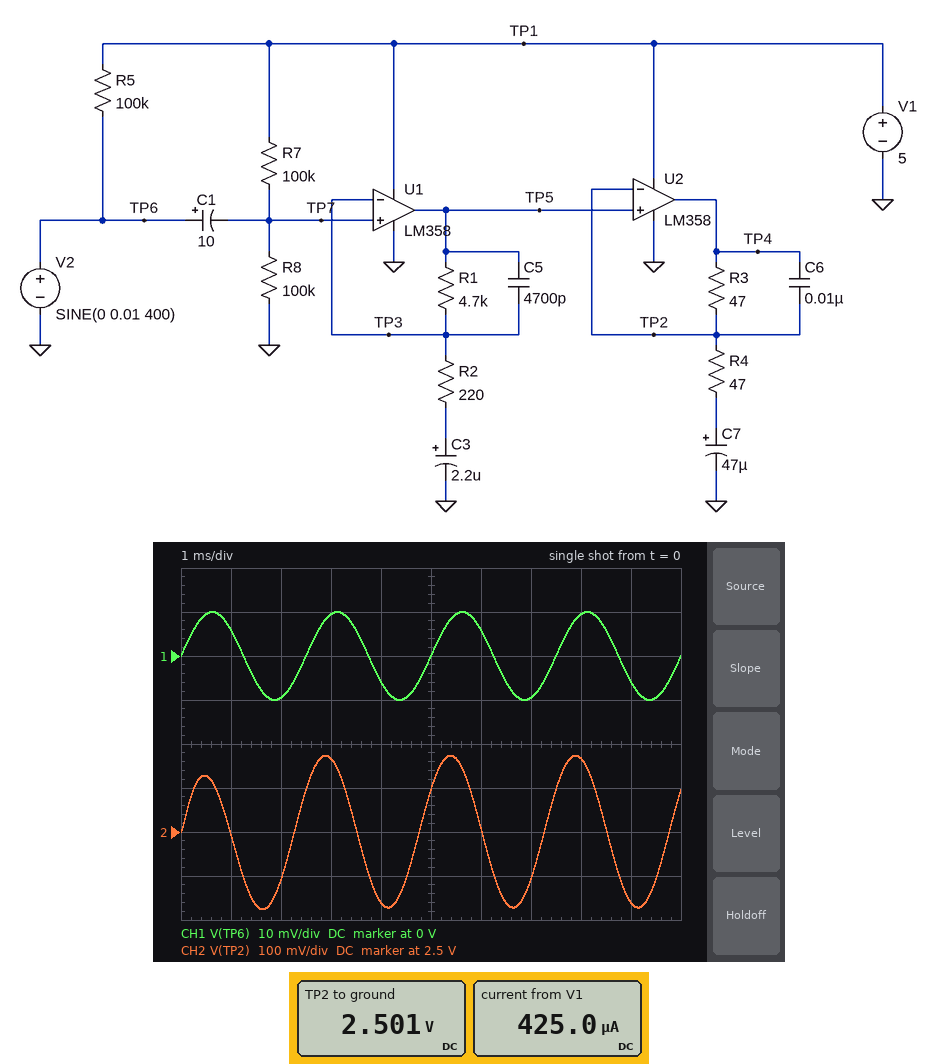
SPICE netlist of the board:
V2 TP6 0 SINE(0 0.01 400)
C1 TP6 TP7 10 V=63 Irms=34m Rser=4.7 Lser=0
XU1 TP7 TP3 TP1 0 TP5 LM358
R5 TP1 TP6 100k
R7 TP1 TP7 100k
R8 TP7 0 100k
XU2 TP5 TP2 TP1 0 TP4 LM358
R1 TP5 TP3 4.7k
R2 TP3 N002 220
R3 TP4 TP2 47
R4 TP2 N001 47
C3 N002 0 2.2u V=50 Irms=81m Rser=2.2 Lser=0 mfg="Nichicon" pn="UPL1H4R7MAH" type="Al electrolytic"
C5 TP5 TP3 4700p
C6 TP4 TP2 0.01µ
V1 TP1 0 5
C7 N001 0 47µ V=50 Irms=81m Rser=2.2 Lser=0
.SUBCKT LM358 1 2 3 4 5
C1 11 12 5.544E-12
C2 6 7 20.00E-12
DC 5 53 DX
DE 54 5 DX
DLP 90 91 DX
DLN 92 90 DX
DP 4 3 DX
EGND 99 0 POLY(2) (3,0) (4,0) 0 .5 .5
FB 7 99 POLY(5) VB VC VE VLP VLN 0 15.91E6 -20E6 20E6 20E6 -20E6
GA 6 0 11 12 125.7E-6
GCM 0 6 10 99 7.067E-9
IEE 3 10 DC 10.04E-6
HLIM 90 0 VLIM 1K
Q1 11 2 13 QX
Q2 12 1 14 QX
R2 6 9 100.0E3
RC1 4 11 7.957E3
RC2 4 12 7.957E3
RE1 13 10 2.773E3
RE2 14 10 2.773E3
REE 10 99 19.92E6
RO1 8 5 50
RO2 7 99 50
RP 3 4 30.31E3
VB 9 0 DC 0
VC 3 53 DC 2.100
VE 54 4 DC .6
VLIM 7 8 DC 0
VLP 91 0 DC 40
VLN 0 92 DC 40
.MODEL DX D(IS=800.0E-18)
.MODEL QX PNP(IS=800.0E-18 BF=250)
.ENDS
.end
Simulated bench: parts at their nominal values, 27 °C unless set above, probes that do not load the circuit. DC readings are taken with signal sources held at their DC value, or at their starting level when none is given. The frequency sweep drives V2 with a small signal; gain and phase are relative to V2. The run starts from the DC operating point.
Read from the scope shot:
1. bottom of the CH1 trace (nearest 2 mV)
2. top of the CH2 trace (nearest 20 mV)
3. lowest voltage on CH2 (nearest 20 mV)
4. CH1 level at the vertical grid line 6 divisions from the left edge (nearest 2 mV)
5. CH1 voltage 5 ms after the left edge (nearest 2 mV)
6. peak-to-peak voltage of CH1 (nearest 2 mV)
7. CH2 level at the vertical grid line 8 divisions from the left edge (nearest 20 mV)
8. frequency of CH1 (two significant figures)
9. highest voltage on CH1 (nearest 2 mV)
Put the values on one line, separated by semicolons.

-10 mV; 2.68 V; 2.32 V; 6 mV; 0 V; 20 mV; 2.66 V; 400 Hz; 10 mV
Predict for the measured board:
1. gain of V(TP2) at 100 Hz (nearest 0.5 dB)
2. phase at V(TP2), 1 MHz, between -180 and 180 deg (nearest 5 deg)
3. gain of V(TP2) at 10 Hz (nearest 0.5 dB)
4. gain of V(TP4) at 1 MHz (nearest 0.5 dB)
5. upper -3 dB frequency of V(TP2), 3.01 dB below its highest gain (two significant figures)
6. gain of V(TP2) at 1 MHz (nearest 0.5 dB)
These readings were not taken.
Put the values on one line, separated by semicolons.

16.5 dB; -165 deg; 1.5 dB; -9.0 dB; 6.8 kHz; -10.0 dB
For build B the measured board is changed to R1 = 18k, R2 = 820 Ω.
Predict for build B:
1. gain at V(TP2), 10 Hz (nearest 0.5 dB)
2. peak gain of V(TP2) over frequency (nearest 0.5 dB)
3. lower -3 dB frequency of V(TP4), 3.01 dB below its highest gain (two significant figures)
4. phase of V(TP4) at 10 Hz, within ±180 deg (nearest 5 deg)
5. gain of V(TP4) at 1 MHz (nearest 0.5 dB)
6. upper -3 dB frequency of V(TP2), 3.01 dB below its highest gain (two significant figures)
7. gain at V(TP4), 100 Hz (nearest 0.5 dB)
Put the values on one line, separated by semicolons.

9.0 dB; 27.0 dB; 100 Hz; 70 deg; -7.5 dB; 2.0 kHz; 29.5 dB
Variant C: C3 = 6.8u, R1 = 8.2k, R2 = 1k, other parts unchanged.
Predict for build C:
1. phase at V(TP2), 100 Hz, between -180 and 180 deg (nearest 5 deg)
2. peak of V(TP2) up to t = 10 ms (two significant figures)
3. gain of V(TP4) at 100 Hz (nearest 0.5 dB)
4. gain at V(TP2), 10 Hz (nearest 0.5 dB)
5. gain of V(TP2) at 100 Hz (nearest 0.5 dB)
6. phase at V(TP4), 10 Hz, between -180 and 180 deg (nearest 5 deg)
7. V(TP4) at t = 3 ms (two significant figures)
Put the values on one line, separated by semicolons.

10 deg; 2.6 V; 23.5 dB; 11.5 dB; 19.0 dB; 60 deg; 2.7 V
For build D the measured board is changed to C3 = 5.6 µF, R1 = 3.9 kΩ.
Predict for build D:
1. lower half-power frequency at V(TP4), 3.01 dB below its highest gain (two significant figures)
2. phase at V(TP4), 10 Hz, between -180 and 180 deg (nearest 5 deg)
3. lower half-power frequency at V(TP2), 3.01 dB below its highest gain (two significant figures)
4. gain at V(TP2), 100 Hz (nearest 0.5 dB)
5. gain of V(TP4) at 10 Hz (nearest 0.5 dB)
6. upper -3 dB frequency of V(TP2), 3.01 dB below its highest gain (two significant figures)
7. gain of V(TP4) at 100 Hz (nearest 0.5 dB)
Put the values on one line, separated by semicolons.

140 Hz; 60 deg; 120 Hz; 21.0 dB; 5.0 dB; 7.8 kHz; 26.0 dB
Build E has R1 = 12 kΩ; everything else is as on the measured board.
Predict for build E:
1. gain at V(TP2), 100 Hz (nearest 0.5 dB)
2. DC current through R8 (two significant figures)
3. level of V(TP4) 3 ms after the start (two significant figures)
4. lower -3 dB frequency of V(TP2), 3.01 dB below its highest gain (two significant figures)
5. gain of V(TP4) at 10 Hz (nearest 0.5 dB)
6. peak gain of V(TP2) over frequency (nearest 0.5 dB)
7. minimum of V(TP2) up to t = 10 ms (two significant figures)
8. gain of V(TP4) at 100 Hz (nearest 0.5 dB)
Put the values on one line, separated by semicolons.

24.0 dB; 25 µA; 3.3 V; 270 Hz; 6.0 dB; 34.0 dB; 2.1 V; 29.0 dB
